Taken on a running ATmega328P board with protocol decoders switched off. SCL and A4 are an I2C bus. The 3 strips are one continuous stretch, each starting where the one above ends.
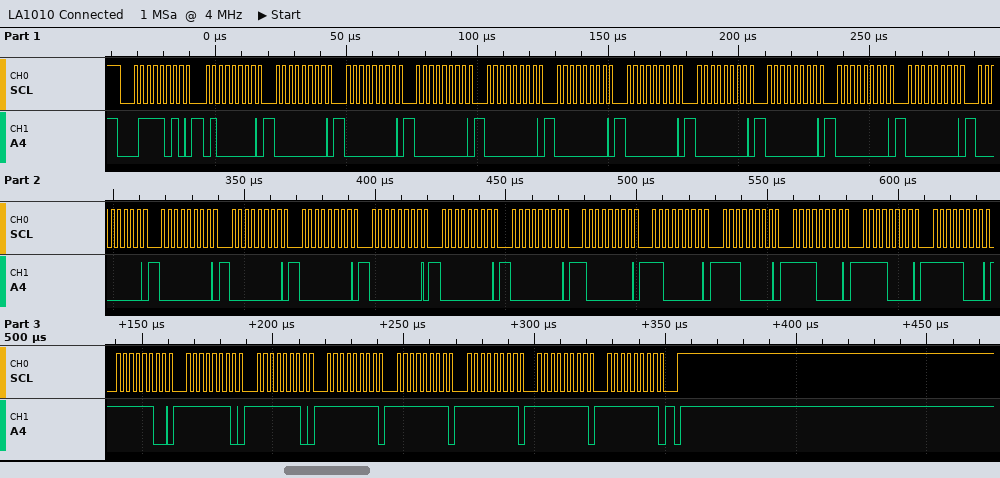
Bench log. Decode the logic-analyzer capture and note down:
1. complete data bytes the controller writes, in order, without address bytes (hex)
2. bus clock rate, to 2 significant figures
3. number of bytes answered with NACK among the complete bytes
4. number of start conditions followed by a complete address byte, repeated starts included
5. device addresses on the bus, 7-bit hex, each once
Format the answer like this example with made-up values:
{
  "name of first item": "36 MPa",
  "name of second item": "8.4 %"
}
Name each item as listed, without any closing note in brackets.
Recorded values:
{
  "complete data bytes the controller writes, in order, without address bytes": "40 00 00 00 00 00 00 00 00 00 00 00 00 00 00 00 00 00 80 C0 E0 F0 F0 F8 FC FE FE FF FF FF FF FF",
  "bus clock rate, to 2 significant figures": "400 kHz",
  "number of bytes answered with NACK among the complete bytes": "0",
  "number of start conditions followed by a complete address byte, repeated starts included": "1",
  "device addresses on the bus, 7-bit hex, each once": "0x3D"
}
